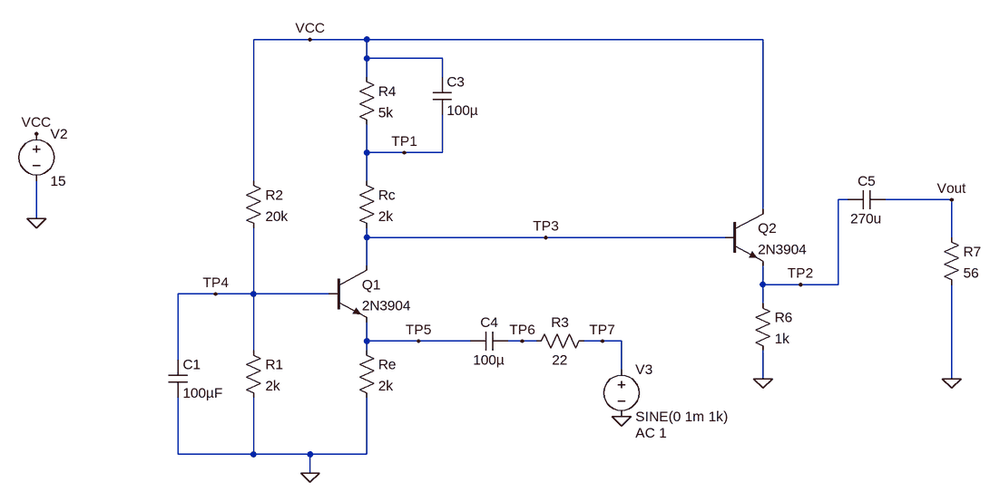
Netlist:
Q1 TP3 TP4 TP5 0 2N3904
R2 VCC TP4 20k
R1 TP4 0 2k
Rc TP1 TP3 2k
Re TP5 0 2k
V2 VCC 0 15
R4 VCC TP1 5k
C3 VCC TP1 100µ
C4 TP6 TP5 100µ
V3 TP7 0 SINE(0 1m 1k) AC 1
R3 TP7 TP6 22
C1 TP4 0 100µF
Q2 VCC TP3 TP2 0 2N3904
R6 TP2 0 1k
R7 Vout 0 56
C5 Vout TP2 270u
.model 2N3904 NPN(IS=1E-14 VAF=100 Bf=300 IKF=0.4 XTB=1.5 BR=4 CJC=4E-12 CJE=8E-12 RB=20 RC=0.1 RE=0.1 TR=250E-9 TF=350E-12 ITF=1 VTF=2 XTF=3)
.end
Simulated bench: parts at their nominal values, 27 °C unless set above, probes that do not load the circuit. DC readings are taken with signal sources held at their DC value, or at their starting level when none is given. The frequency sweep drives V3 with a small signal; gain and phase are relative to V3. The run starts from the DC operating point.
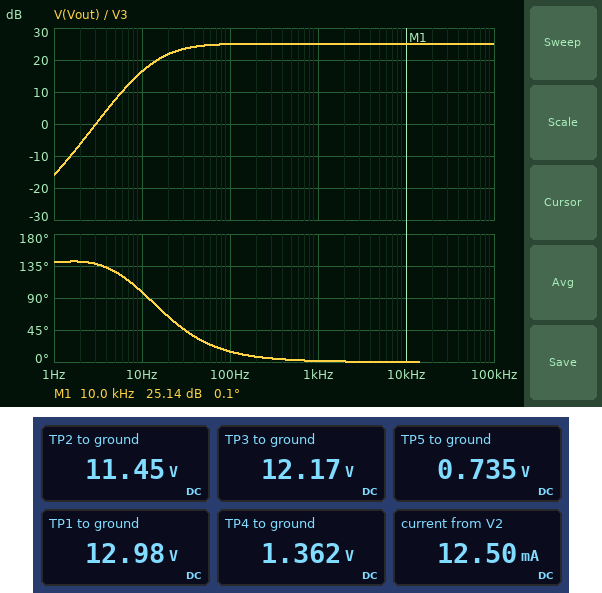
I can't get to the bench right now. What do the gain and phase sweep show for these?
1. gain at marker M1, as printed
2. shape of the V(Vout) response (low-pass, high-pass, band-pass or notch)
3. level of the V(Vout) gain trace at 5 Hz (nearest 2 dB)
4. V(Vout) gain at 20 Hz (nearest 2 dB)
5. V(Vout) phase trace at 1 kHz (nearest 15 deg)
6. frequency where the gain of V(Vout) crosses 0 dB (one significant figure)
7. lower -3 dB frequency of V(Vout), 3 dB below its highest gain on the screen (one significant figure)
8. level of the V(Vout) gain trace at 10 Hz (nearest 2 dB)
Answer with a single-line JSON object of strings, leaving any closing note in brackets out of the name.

{"gain at marker M1, as printed": "25.14 dB", "shape of the V(Vout) response": "high-pass", "level of the V(Vout) gain trace at 5 Hz": "8 dB", "V(Vout) gain at 20 Hz": "22 dB", "V(Vout) phase trace at 1 kHz": "0 deg", "frequency where the gain of V(Vout) crosses 0 dB": "3 Hz", "lower -3 dB frequency of V(Vout), 3 dB below its highest gain on the screen": "20 Hz", "level of the V(Vout) gain trace at 10 Hz": "16 dB"}
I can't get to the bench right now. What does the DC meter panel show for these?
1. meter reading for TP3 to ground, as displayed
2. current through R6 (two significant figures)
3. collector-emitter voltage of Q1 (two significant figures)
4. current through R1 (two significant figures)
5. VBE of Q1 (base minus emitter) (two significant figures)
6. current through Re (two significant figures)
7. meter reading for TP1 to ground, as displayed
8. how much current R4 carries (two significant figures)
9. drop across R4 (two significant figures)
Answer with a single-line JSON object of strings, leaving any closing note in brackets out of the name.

{"meter reading for TP3 to ground, as displayed": "12.17 V", "current through R6": "11 mA", "collector-emitter voltage of Q1": "11 V", "current through R1": "680 µA", "VBE of Q1 (base minus emitter)": "630 mV", "current through Re": "370 µA", "meter reading for TP1 to ground, as displayed": "12.98 V", "how much current R4 carries": "400 µA", "drop across R4": "2.0 V"}
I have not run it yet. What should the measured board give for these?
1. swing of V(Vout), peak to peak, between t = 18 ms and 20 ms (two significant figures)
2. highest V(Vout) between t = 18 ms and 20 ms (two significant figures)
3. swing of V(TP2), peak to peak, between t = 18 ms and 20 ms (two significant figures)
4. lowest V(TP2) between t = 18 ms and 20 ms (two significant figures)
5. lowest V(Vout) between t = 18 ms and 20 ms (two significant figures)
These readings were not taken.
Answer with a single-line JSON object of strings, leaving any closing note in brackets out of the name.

{"swing of V(Vout), peak to peak, between t = 18 ms and 20 ms": "36 mV", "highest V(Vout) between t = 18 ms and 20 ms": "18 mV", "swing of V(TP2), peak to peak, between t = 18 ms and 20 ms": "36 mV", "lowest V(TP2) between t = 18 ms and 20 ms": "11 V", "lowest V(Vout) between t = 18 ms and 20 ms": "-18 mV"}
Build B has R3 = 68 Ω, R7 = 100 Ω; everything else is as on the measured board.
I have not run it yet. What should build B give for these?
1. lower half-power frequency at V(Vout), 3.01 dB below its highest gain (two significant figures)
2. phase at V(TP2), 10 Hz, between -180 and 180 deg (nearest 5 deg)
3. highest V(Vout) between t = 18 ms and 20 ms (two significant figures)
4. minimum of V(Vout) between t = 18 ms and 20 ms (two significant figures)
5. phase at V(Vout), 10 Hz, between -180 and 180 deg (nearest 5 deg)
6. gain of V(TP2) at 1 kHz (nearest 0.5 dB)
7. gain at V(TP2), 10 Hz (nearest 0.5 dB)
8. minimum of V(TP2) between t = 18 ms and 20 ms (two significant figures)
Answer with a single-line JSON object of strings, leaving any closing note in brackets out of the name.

{"lower half-power frequency at V(Vout), 3.01 dB below its highest gain": "14 Hz", "phase at V(TP2), 10 Hz, between -180 and 180 deg": "45 deg", "highest V(Vout) between t = 18 ms and 20 ms": "13 mV", "minimum of V(Vout) between t = 18 ms and 20 ms": "-13 mV", "phase at V(Vout), 10 Hz, between -180 and 180 deg": "75 deg", "gain of V(TP2) at 1 kHz": "22.0 dB", "gain at V(TP2), 10 Hz": "18.5 dB", "minimum of V(TP2) between t = 18 ms and 20 ms": "11 V"}
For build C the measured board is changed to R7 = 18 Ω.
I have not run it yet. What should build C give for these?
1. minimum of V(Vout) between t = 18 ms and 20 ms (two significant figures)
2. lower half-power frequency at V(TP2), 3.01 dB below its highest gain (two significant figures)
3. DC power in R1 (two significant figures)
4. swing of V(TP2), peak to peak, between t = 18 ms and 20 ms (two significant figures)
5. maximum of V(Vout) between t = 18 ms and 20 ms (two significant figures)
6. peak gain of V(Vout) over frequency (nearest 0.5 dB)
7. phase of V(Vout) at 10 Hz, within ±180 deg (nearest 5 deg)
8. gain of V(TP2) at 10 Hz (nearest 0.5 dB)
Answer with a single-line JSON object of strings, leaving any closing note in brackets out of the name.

{"minimum of V(Vout) between t = 18 ms and 20 ms": "-14 mV", "lower half-power frequency at V(TP2), 3.01 dB below its highest gain": "11 Hz", "DC power in R1": "930 µW", "swing of V(TP2), peak to peak, between t = 18 ms and 20 ms": "28 mV", "maximum of V(Vout) between t = 18 ms and 20 ms": "14 mV", "peak gain of V(Vout) over frequency": "23.0 dB", "phase of V(Vout) at 10 Hz, within ±180 deg": "120 deg", "gain of V(TP2) at 10 Hz": "20.0 dB"}
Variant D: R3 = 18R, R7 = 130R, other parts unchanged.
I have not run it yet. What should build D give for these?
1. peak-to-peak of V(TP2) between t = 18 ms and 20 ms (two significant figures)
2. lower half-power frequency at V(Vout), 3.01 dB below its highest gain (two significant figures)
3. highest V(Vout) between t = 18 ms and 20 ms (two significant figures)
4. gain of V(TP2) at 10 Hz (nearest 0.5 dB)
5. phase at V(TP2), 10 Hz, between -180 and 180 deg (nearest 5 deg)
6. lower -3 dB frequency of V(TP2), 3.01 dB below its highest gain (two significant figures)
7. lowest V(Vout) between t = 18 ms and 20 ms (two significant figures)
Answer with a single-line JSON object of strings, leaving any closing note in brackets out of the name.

{"peak-to-peak of V(TP2) between t = 18 ms and 20 ms": "41 mV", "lower half-power frequency at V(Vout), 3.01 dB below its highest gain": "19 Hz", "highest V(Vout) between t = 18 ms and 20 ms": "20 mV", "gain of V(TP2) at 10 Hz": "20.0 dB", "phase at V(TP2), 10 Hz, between -180 and 180 deg": "55 deg", "lower -3 dB frequency of V(TP2), 3.01 dB below its highest gain": "18 Hz", "lowest V(Vout) between t = 18 ms and 20 ms": "-21 mV"}
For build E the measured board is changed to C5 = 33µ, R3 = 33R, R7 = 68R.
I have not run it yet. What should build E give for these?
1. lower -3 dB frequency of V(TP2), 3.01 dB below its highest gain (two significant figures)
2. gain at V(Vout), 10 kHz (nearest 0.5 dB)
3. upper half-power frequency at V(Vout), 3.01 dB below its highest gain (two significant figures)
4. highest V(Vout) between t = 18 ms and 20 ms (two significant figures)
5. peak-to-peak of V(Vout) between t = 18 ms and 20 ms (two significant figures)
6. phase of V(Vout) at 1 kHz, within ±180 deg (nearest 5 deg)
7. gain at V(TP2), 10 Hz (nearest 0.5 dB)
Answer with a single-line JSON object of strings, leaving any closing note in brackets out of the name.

{"lower -3 dB frequency of V(TP2), 3.01 dB below its highest gain": "13 Hz", "gain at V(Vout), 10 kHz": "24.5 dB", "upper half-power frequency at V(Vout), 3.01 dB below its highest gain": "8.6 MHz", "highest V(Vout) between t = 18 ms and 20 ms": "16 mV", "peak-to-peak of V(Vout) between t = 18 ms and 20 ms": "33 mV", "phase of V(Vout) at 1 kHz, within ±180 deg": "5 deg", "gain at V(TP2), 10 Hz": "20.0 dB"}
